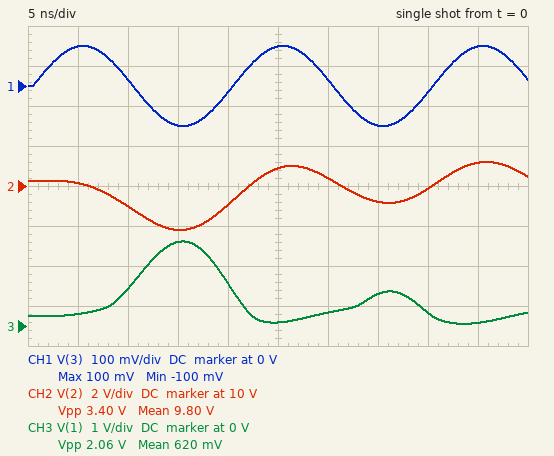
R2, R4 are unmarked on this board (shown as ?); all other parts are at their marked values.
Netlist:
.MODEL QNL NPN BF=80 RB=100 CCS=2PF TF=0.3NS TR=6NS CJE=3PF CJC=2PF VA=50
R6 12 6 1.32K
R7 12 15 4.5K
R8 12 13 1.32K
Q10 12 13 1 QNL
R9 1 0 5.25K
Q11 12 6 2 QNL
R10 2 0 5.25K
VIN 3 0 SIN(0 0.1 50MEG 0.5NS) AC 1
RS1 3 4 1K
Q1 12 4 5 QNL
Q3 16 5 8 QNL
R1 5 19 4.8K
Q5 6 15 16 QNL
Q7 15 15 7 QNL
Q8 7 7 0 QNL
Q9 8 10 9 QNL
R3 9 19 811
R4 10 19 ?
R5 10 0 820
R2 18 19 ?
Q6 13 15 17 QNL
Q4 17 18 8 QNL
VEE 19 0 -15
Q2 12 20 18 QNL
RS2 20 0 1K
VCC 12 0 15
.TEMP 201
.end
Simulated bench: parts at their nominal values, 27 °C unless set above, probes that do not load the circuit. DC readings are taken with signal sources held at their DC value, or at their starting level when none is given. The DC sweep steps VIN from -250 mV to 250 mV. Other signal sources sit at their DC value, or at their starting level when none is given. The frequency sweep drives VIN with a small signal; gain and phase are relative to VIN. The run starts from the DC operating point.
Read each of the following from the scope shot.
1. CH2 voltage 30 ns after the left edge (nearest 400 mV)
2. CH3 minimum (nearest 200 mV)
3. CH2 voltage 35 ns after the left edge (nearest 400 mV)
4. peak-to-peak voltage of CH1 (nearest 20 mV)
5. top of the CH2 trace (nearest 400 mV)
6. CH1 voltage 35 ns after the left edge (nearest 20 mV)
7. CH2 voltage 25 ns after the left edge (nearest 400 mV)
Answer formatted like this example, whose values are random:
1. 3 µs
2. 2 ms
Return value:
1. 10.4 V
2. 0 V
3. 9.2 V
4. 200 mV
5. 11.2 V
6. -100 mV
7. 10.8 V
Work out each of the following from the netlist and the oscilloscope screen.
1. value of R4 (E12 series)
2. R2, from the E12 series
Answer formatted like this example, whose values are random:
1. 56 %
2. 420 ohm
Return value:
1. 4.7 kΩ
2. 15 kΩ
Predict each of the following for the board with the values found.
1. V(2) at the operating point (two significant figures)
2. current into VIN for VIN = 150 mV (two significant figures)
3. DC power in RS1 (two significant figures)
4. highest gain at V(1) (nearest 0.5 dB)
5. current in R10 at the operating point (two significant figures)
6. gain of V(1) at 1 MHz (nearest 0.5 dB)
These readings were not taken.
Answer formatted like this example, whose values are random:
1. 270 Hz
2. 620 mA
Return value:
1. 10 V
2. -30 µA
3. 840 nW
4. 20.5 dB
5. 2.0 mA
6. 20.5 dB
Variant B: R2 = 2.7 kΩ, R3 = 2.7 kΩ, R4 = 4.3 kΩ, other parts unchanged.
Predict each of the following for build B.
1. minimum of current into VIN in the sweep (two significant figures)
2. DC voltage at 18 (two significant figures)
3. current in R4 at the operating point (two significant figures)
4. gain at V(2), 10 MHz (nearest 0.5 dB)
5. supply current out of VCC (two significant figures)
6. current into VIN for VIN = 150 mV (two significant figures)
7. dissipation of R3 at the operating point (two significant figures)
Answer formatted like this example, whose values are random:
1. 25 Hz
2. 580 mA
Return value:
1. -30 µA
2. -640 mV
3. 2.9 mA
4. 27.5 dB
5. 20 mA
6. -29 µA
7. 53 mW
